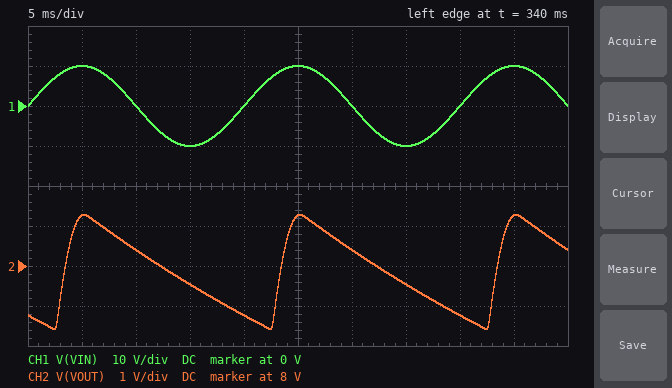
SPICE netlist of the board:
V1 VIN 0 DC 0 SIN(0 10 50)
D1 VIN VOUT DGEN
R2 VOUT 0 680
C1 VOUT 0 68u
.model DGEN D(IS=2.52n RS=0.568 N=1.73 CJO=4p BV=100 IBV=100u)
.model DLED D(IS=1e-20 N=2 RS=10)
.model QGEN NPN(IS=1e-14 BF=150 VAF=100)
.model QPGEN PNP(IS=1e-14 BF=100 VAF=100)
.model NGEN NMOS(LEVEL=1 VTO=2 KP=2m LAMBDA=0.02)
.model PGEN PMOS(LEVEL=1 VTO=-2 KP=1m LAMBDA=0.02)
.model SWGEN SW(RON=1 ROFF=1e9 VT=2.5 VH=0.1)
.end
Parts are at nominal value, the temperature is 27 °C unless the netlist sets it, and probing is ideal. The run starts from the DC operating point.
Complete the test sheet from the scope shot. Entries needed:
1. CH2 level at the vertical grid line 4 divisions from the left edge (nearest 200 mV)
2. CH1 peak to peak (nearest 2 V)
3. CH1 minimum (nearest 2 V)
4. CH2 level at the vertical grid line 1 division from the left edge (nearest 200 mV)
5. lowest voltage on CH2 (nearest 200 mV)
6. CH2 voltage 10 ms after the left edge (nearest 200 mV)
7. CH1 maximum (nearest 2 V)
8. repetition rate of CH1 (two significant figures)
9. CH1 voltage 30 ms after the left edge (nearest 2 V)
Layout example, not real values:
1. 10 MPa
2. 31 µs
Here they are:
1. 6.8 V
2. 20 V
3. -10 V
4. 9.2 V
5. 6.4 V
6. 8.4 V
7. 10 V
8. 50 Hz
9. 0 V
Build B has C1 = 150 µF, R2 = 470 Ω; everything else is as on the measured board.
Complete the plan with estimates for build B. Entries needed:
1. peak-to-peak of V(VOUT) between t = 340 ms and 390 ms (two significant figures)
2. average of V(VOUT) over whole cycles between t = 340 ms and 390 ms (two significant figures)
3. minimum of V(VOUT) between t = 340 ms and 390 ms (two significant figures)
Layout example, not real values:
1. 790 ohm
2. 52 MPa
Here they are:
1. 2.0 V
2. 8.2 V
3. 7.2 V
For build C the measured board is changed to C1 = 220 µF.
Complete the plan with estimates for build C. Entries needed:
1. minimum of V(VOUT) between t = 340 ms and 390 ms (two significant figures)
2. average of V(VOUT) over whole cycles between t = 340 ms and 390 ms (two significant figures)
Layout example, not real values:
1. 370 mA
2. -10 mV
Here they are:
1. 8.2 V
2. 8.7 V
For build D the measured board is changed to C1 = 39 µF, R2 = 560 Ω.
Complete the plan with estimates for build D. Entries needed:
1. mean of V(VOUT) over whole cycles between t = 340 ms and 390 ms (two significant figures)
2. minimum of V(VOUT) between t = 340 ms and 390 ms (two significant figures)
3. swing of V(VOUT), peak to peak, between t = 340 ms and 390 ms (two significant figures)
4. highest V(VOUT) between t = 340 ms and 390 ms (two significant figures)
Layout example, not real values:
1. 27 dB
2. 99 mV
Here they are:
1. 6.8 V
2. 4.4 V
3. 4.9 V
4. 9.3 V
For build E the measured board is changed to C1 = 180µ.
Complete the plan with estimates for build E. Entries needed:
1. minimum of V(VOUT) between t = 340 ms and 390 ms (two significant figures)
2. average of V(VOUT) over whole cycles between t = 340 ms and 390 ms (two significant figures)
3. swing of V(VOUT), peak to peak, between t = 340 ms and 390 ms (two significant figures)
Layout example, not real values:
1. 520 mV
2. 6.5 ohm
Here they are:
1. 8.0 V
2. 8.6 V
3. 1.3 V
